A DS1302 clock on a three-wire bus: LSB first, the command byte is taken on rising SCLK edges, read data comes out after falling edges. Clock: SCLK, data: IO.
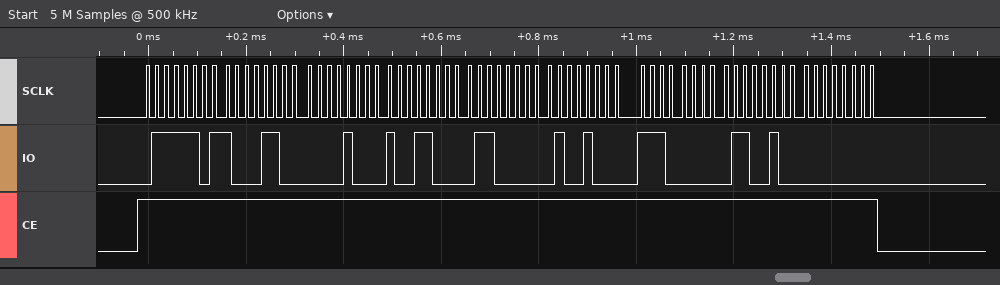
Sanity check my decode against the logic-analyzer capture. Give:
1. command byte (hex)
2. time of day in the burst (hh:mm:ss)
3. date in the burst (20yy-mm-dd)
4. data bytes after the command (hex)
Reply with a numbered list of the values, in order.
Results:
1. 0xBE
2. 19:10:31
3. 2026-12-06
4. 31 10 19 06 12 07 26 00
